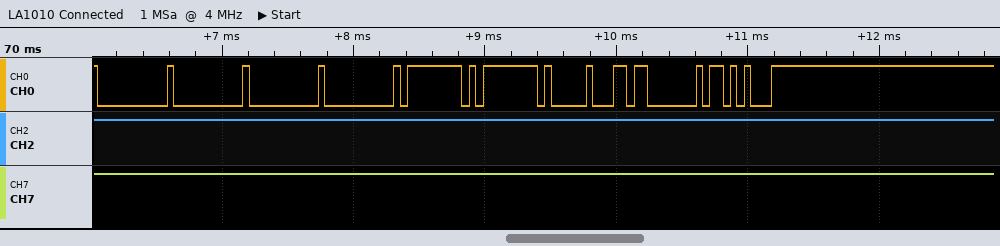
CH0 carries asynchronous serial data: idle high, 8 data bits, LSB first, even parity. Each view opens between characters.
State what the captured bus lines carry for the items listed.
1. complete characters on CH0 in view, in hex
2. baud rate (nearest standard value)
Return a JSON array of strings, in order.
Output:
["00, 00, 00, 00, FF, FF, 10, 03, 2B", "19200 baud"]
